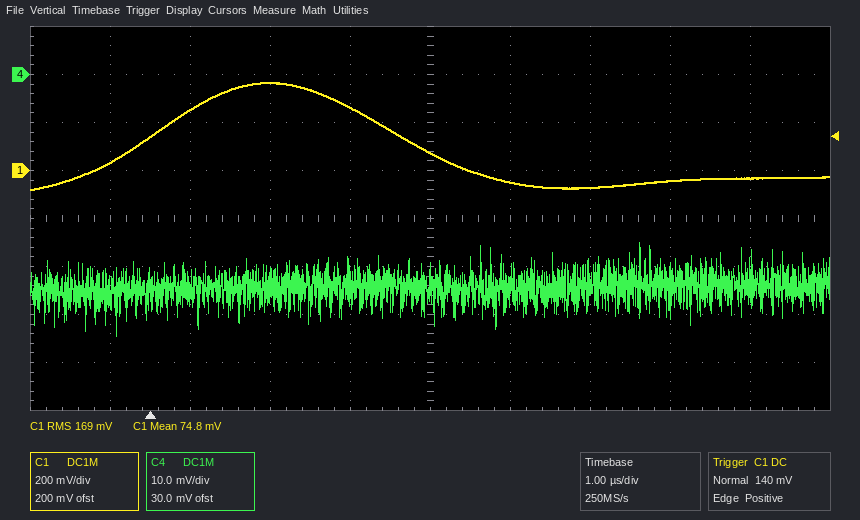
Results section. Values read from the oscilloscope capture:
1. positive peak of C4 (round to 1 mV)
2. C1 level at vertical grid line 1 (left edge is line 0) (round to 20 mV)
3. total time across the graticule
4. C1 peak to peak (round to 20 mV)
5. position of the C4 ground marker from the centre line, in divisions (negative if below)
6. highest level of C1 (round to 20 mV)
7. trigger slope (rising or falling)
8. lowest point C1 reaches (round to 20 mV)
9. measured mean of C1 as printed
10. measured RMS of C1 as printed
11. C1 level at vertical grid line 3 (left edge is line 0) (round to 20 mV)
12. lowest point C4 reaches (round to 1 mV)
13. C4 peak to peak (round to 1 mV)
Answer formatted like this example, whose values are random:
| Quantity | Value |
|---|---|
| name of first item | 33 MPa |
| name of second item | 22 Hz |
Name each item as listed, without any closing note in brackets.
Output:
| Quantity | Value |
|---|---|
| positive peak of C4 | -35 mV |
| C1 level at vertical grid line 1 (left edge is line 0) | 40 mV |
| total time across the graticule | 10 µs |
| C1 peak to peak | 440 mV |
| position of the C4 ground marker from the centre line, in divisions | +3.0 div |
| highest level of C1 | 360 mV |
| trigger slope | rising |
| lowest point C1 reaches | -80 mV |
| measured mean of C1 as printed | 74.8 mV |
| measured RMS of C1 as printed | 169 mV |
| C1 level at vertical grid line 3 (left edge is line 0) | 360 mV |
| lowest point C4 reaches | -54 mV |
| C4 peak to peak | 19 mV |
